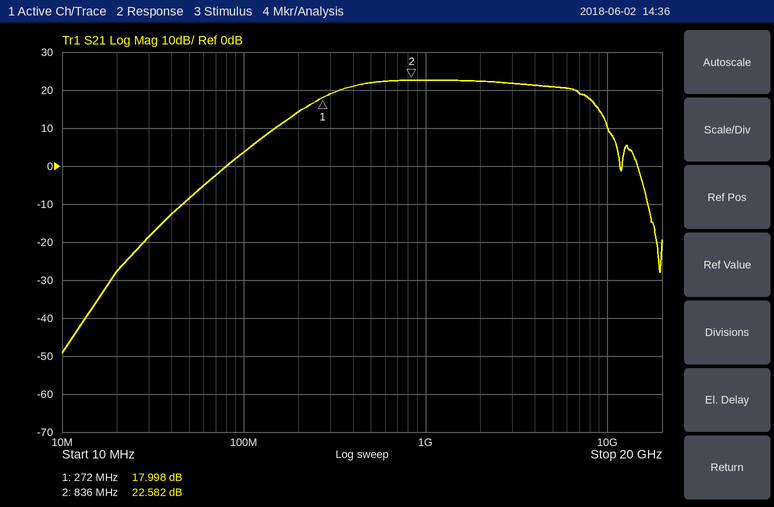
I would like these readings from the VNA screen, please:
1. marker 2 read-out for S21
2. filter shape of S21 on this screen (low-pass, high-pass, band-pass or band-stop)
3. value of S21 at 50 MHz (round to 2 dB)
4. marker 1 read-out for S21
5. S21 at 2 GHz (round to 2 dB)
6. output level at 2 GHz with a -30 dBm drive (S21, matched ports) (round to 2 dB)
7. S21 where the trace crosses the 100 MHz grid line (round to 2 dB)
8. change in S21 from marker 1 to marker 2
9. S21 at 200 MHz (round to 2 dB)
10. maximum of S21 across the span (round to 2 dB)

22.582 dB
band-pass
-8 dB
17.998 dB
22 dB
-8 dBm
4 dB
4.584 dB
14 dB
22 dB
